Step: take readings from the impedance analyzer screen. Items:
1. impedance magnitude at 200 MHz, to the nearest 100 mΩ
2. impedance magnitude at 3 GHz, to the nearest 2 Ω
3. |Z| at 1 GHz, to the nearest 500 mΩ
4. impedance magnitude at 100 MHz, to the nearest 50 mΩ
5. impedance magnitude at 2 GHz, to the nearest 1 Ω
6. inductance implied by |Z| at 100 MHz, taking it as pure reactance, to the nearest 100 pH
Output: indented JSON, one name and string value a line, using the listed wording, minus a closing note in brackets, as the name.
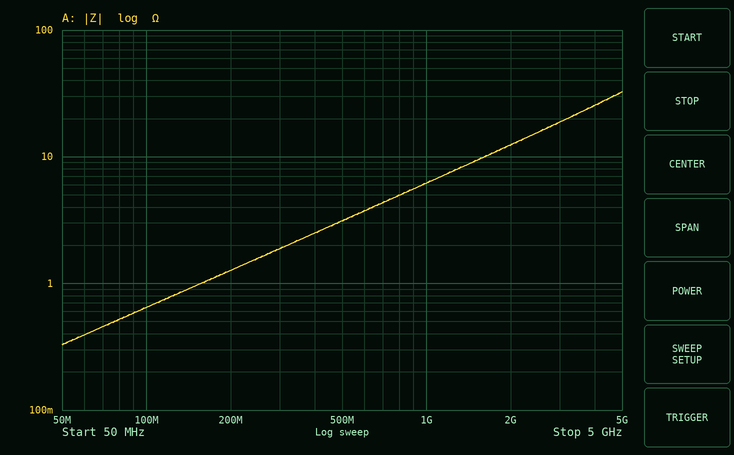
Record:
{
  "impedance magnitude at 200 MHz, to the nearest 100 mΩ": "1.3 Ω",
  "impedance magnitude at 3 GHz, to the nearest 2 Ω": "18 Ω",
  "|Z| at 1 GHz, to the nearest 500 mΩ": "6.0 Ω",
  "impedance magnitude at 100 MHz, to the nearest 50 mΩ": "650 mΩ",
  "impedance magnitude at 2 GHz, to the nearest 1 Ω": "12 Ω",
  "inductance implied by |Z| at 100 MHz, taking it as pure reactance, to the nearest 100 pH": "1.0 nH"
}
